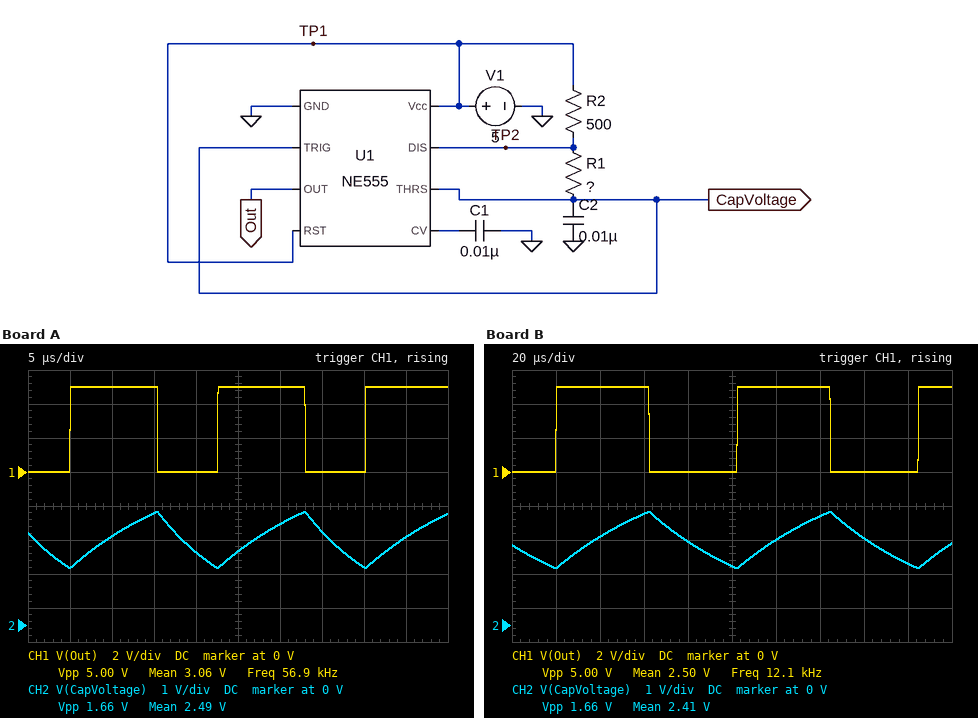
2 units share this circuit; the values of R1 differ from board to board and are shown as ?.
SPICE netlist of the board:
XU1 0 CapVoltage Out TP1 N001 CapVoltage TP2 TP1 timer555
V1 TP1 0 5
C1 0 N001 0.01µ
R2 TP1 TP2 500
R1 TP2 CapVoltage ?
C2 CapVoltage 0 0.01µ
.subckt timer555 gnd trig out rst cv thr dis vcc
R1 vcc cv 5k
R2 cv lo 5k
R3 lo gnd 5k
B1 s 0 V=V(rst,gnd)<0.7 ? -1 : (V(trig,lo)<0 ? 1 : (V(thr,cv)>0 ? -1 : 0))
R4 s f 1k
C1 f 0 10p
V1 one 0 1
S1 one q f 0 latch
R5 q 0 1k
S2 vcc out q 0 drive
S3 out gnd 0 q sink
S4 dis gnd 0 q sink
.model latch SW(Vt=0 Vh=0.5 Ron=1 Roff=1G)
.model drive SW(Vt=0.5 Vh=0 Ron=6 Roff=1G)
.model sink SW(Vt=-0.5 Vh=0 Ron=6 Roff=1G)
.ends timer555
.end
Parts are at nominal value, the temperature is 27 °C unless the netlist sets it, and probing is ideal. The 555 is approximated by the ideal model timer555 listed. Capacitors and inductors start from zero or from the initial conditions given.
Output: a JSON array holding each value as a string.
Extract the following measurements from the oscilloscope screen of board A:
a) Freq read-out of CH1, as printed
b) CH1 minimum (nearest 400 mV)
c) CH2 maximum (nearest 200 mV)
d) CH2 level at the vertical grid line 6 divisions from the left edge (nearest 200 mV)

["56.9 kHz", "0 V", "3.4 V", "3.0 V"]
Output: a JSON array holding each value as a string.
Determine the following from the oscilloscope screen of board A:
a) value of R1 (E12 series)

["1 kΩ"]
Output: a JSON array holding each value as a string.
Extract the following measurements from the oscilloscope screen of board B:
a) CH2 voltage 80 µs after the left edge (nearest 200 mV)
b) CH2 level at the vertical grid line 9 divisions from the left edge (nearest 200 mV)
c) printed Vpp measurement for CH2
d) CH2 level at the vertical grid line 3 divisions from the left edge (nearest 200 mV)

["2.4 V", "1.8 V", "1.66 V", "3.2 V"]
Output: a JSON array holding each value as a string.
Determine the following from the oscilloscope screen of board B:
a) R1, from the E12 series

["5.6 kΩ"]
